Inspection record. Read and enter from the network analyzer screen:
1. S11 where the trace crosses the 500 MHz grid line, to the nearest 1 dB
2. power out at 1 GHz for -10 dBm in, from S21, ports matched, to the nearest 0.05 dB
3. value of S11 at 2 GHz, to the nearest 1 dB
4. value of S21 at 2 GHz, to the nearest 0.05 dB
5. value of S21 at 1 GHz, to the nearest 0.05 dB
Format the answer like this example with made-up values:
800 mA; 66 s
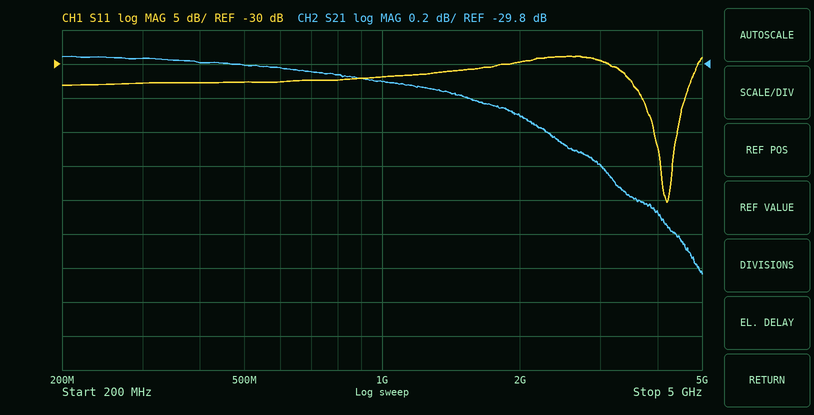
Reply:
-33 dB; -39.90 dBm; -30 dB; -30.10 dB; -29.90 dB
